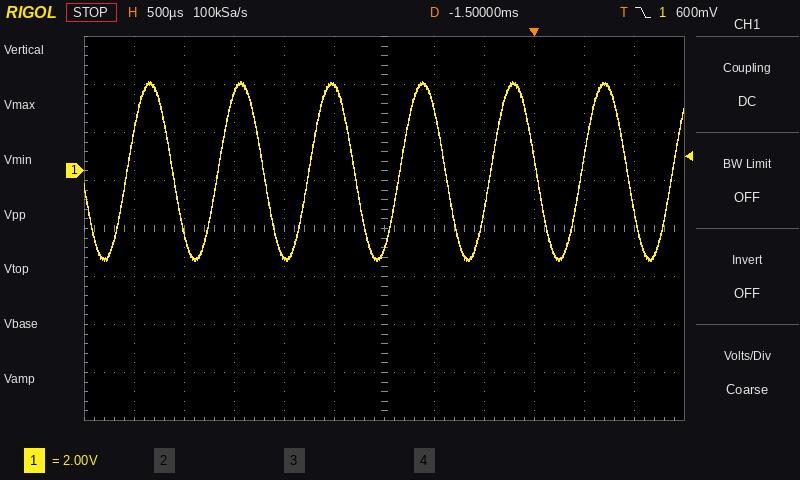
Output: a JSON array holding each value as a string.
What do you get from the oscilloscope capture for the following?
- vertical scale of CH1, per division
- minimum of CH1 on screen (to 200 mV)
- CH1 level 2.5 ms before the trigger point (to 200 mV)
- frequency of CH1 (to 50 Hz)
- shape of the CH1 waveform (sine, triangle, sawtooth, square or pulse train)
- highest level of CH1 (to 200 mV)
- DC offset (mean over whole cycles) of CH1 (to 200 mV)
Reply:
["2 V", "-3.8 V", "-3.6 V", "1.10 kHz", "sine", "3.8 V", "0.0 V"]
